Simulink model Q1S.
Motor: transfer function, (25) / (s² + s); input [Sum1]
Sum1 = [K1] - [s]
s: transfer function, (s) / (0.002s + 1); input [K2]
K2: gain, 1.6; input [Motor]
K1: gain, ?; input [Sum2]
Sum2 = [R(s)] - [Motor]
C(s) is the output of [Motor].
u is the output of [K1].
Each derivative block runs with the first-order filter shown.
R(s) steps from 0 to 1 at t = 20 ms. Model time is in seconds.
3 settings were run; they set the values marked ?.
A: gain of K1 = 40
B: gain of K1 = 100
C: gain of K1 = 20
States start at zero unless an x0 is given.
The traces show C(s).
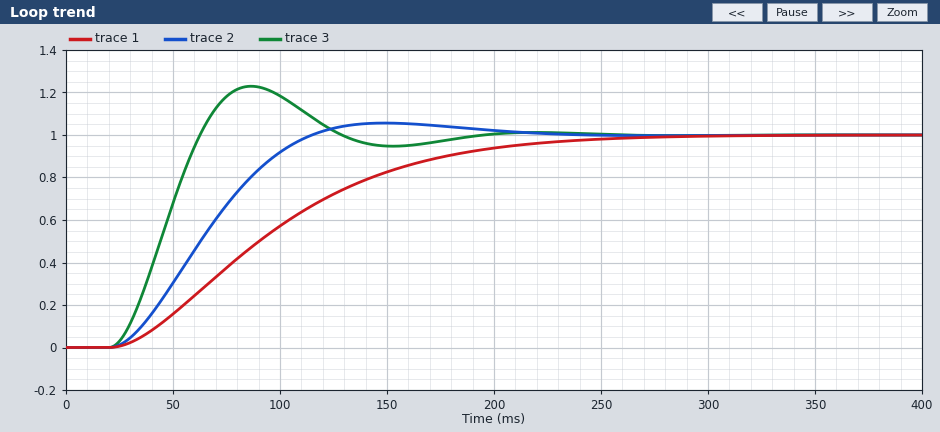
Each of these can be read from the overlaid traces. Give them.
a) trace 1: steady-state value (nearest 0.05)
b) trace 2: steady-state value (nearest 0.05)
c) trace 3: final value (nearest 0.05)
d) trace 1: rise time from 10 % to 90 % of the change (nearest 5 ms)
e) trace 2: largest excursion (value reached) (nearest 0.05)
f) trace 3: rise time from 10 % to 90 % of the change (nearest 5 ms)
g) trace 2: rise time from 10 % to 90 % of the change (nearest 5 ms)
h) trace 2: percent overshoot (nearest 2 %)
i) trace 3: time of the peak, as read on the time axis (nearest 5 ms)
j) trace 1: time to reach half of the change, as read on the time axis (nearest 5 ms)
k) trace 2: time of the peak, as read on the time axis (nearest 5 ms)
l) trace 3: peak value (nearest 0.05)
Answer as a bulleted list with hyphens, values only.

- 1.00
- 1.00
- 1.00
- 135 ms
- 1.05
- 30 ms
- 60 ms
- 6 %
- 85 ms
- 90 ms
- 150 ms
- 1.25
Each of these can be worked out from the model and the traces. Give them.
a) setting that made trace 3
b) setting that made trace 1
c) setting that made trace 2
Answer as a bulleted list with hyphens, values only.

- B
- C
- A
